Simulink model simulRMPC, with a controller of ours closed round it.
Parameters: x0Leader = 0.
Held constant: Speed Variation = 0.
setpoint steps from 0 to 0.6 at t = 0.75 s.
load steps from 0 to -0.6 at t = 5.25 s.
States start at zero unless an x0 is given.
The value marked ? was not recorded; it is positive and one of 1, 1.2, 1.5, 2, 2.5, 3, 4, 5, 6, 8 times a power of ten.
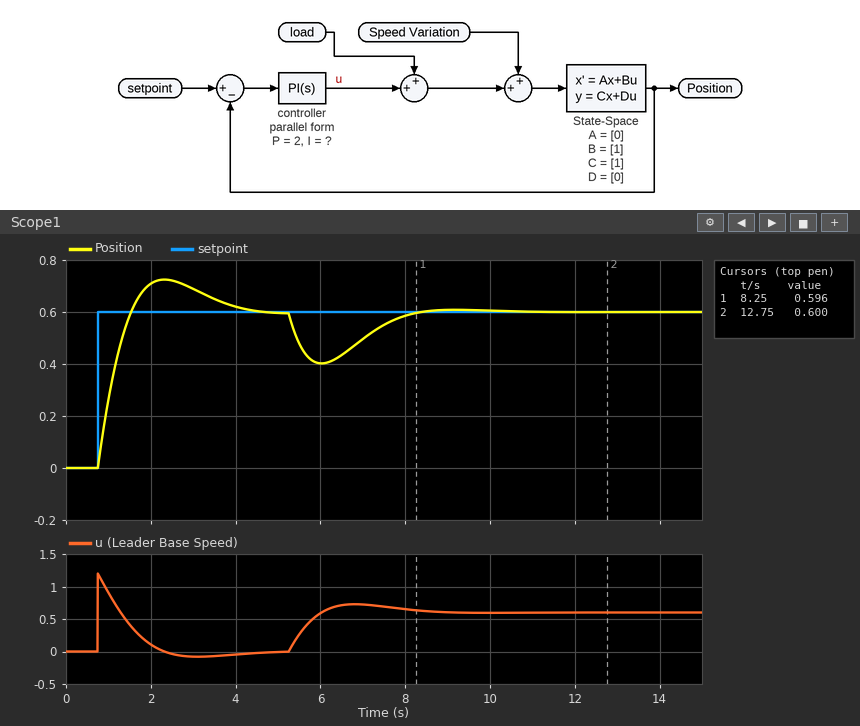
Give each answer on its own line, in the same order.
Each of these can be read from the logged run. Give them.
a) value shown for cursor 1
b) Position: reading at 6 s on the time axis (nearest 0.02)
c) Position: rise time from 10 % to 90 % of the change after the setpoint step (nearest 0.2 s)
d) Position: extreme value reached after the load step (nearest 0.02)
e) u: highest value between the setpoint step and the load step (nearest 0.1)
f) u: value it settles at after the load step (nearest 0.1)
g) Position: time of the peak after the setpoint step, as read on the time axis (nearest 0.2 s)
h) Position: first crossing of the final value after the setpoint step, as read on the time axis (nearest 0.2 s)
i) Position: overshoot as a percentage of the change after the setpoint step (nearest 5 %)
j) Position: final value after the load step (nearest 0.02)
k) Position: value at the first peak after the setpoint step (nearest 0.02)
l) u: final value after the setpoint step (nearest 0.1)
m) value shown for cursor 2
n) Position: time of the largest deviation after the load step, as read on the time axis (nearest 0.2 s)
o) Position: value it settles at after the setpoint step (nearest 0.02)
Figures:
0.596
0.40
0.6 s
0.40
1.2
0.6
2.4 s
1.6 s
20 %
0.60
0.72
0.0
0.600
6.0 s
0.60
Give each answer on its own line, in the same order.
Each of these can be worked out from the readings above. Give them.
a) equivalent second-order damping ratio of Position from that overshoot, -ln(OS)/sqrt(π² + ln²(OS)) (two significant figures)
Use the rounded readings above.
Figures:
0.46
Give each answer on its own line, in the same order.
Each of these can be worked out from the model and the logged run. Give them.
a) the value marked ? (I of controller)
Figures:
2
